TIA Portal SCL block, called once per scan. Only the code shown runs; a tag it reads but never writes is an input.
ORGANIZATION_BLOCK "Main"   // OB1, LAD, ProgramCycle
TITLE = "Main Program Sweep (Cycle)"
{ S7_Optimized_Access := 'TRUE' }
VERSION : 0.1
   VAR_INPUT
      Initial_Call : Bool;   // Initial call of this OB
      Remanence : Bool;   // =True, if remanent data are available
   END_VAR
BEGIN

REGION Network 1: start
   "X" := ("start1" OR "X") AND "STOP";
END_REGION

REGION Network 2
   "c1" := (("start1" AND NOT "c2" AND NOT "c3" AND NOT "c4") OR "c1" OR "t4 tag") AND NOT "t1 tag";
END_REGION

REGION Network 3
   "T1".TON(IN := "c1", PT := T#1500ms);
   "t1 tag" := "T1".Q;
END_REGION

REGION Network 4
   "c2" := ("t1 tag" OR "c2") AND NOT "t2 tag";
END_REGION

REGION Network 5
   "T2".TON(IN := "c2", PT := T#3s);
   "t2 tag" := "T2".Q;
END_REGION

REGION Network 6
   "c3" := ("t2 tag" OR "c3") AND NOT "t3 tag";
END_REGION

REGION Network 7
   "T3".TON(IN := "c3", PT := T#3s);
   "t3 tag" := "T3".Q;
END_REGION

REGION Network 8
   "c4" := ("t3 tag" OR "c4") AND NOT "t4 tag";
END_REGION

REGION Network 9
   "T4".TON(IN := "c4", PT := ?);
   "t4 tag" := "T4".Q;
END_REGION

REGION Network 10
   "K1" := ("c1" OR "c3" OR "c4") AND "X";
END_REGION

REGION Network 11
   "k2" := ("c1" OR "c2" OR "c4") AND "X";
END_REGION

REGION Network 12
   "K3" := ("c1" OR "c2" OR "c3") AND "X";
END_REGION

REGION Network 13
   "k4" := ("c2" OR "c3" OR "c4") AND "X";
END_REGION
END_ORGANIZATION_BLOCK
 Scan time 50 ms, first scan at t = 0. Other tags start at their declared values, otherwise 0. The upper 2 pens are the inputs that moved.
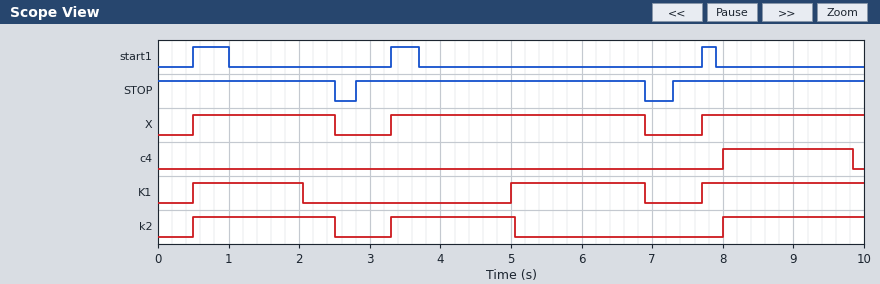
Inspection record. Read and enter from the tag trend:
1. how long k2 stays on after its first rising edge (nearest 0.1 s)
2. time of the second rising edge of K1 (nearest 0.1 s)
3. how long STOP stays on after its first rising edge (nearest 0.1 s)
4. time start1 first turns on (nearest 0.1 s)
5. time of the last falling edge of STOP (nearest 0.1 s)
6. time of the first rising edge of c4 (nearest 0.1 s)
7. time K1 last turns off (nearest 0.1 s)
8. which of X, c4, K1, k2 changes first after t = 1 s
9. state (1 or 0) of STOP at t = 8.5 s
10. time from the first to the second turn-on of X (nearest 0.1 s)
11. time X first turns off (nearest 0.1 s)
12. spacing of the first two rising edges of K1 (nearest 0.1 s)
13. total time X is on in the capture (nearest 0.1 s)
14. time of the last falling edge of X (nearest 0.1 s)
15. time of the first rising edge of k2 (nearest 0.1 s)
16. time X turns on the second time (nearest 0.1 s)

2.0 s
5.0 s
4.1 s
0.5 s
6.9 s
8.0 s
6.9 s
K1
1
2.8 s
2.5 s
4.5 s
7.9 s
6.9 s
0.5 s
3.3 s
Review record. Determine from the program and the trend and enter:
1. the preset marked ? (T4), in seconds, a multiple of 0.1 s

1.8 s
